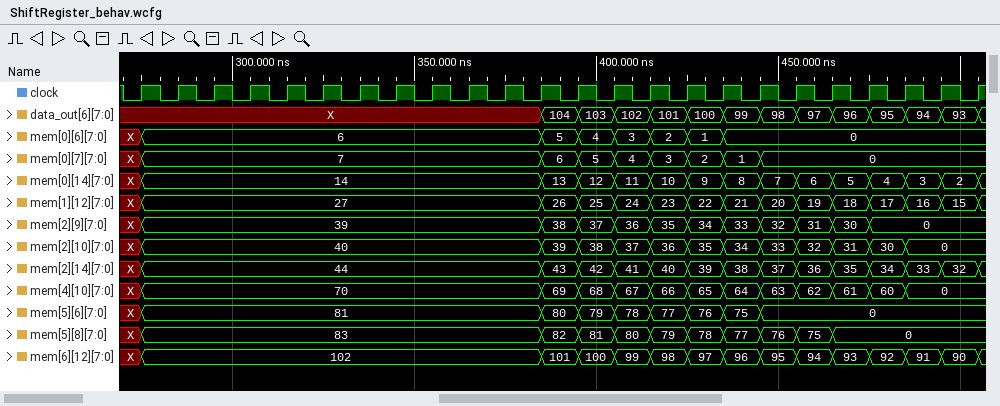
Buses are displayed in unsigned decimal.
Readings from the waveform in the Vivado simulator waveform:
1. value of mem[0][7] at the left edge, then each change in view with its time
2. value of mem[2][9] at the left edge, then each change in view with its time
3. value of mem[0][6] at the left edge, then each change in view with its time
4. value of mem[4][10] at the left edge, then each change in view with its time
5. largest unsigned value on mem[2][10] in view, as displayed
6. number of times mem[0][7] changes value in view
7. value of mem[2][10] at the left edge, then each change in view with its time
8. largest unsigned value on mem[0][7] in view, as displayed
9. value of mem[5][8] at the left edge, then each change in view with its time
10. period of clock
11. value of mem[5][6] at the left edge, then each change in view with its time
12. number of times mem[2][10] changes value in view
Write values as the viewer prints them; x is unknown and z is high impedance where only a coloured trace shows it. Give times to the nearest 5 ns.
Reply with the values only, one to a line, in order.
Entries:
X, 7 at 275 ns, 6 at 385 ns, 5 at 395 ns, 4 at 405 ns, 3 at 415 ns, 2 at 425 ns, 1 at 435 ns, 0 at 445 ns
X, 39 at 275 ns, 38 at 385 ns, 37 at 395 ns, 36 at 405 ns, 35 at 415 ns, 34 at 425 ns, 33 at 435 ns, 32 at 445 ns, 31 at 455 ns, 30 at 465 ns, 0 at 475 ns
X, 6 at 275 ns, 5 at 385 ns, 4 at 395 ns, 3 at 405 ns, 2 at 415 ns, 1 at 425 ns, 0 at 435 ns
X, 70 at 275 ns, 69 at 385 ns, 68 at 395 ns, 67 at 405 ns, 66 at 415 ns, 65 at 425 ns, 64 at 435 ns, 63 at 445 ns, 62 at 455 ns, 61 at 465 ns, 60 at 475 ns, 0 at 485 ns
40
8
X, 40 at 275 ns, 39 at 385 ns, 38 at 395 ns, 37 at 405 ns, 36 at 415 ns, 35 at 425 ns, 34 at 435 ns, 33 at 445 ns, 32 at 455 ns, 31 at 465 ns, 30 at 475 ns, 0 at 485 ns
7
X, 83 at 275 ns, 82 at 385 ns, 81 at 395 ns, 80 at 405 ns, 79 at 415 ns, 78 at 425 ns, 77 at 435 ns, 76 at 445 ns, 75 at 455 ns, 0 at 465 ns
10 ns
X, 81 at 275 ns, 80 at 385 ns, 79 at 395 ns, 78 at 405 ns, 77 at 415 ns, 76 at 425 ns, 75 at 435 ns, 0 at 445 ns
12
